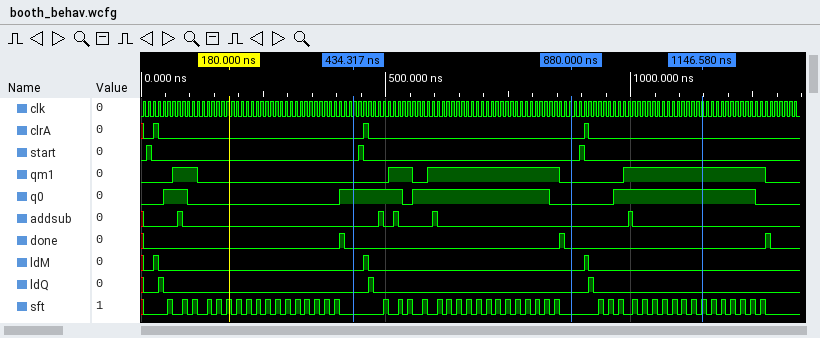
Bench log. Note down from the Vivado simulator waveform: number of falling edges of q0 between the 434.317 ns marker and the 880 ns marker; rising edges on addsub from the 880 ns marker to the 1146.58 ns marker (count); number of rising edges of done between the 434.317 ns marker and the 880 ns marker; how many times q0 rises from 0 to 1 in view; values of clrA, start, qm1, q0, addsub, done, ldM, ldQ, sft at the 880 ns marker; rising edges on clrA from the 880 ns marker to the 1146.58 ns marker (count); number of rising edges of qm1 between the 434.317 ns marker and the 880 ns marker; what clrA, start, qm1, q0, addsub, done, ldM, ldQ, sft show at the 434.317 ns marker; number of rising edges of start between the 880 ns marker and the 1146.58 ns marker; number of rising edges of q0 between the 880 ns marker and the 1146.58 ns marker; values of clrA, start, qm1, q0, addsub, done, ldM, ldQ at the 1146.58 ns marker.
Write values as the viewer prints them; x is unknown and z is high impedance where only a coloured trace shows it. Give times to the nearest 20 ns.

2
1
1
4
clrA=0, start=0, qm1=0, q0=0, addsub=0, done=0, ldM=0, ldQ=0, sft=0
1
2
clrA=0, start=0, qm1=0, q0=1, addsub=0, done=0, ldM=0, ldQ=0, sft=0
1
1
clrA=0, start=0, qm1=1, q0=1, addsub=0, done=0, ldM=0, ldQ=0
